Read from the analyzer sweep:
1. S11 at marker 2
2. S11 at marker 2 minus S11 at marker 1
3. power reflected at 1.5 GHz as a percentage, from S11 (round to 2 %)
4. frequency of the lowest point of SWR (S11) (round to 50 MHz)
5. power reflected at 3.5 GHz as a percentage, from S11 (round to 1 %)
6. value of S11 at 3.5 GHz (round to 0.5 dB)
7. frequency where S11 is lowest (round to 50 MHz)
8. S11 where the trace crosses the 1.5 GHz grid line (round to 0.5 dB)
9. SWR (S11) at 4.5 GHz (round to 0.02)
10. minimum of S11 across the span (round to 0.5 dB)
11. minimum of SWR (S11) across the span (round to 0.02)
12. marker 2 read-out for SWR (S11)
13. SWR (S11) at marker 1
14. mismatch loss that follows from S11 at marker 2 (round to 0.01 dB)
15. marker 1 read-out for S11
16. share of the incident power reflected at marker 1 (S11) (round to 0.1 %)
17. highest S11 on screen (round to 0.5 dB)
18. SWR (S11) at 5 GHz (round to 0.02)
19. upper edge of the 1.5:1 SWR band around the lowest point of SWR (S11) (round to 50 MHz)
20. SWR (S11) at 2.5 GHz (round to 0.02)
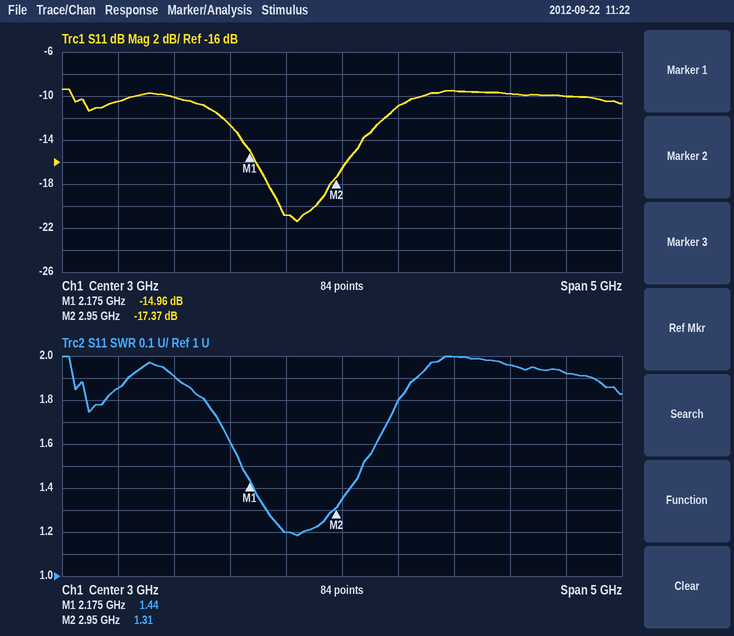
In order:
-17.37 dB
-2.41 dB
10 %
2.60 GHz
8 %
-11.0 dB
2.60 GHz
-10.0 dB
1.96
-21.5 dB
1.18
1.31
1.44
0.08 dB
-14.96 dB
3.2 %
-9.5 dB
1.92
3.20 GHz
1.20
